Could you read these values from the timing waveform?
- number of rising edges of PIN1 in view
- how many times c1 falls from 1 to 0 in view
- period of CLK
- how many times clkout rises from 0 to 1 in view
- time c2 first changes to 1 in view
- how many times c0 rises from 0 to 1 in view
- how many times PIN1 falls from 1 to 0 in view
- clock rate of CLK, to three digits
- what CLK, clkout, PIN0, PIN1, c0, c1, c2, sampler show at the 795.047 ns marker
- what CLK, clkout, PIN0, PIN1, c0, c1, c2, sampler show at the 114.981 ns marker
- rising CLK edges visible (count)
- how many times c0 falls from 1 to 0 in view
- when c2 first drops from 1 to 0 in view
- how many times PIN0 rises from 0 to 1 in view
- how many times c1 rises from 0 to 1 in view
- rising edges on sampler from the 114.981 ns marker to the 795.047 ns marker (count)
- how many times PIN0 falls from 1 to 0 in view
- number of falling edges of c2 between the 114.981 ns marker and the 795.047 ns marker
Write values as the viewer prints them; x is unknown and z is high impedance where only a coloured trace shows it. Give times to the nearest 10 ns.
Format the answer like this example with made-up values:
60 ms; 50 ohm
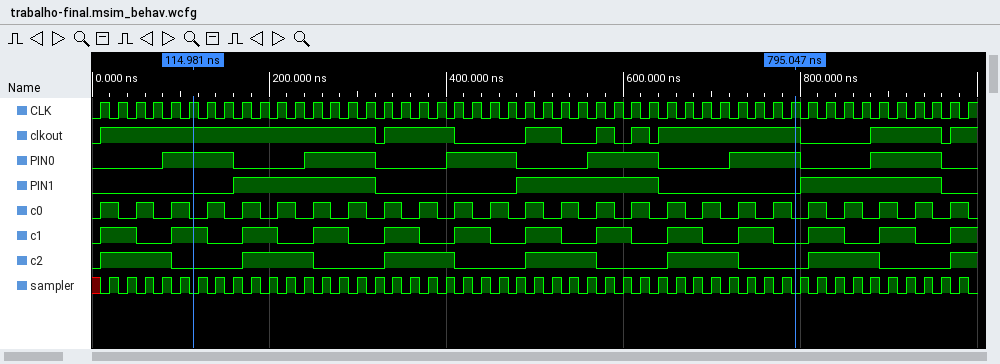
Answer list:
3; 12; 20 ns; 8; 10 ns; 25; 3; 50.0 MHz; CLK=1, clkout=1, PIN0=1, PIN1=0, c0=0, c1=0, c2=0, sampler=0; CLK=1, clkout=1, PIN0=1, PIN1=0, c0=0, c1=1, c2=0, sampler=0; 50; 25; 90 ns; 6; 13; 34; 6; 4
